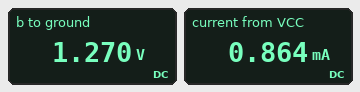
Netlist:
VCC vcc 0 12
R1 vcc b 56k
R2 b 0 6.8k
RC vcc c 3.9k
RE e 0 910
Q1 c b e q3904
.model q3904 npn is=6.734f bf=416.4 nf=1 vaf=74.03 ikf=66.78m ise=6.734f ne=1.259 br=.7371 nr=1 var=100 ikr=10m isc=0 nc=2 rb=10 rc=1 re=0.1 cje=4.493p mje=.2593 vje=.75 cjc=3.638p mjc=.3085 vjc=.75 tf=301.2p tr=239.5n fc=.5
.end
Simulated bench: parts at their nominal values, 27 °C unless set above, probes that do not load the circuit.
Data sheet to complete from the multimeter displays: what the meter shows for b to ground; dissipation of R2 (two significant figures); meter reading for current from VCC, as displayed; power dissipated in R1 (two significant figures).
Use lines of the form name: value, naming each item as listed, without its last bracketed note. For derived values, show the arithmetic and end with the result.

what the meter shows for b to ground: 1.270 V
dissipation of R2: (1.27 V)^2 / 6.8 kΩ = 240 µW
meter reading for current from VCC, as displayed: 0.864 mA
power dissipated in R1: (12 V - 1.27 V)^2 / 56 kΩ = 2.1 mW
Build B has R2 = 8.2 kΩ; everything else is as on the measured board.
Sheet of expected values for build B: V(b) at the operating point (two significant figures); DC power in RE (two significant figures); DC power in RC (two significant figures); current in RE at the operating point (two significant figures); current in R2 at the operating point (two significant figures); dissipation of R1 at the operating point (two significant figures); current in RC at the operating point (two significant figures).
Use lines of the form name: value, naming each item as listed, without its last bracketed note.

V(b) at the operating point: 1.5 V
DC power in RE: 750 µW
DC power in RC: 3.2 mW
current in RE at the operating point: 910 µA
current in R2 at the operating point: 180 µA
dissipation of R1 at the operating point: 2.0 mW
current in RC at the operating point: 900 µA
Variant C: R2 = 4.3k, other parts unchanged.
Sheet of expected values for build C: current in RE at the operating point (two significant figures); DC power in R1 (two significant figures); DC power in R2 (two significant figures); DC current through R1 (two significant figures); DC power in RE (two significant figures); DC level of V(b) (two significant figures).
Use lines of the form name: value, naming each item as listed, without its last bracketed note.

current in RE at the operating point: 240 µA
DC power in R1: 2.2 mW
DC power in R2: 170 µW
DC current through R1: 200 µA
DC power in RE: 54 µW
DC level of V(b): 850 mV
